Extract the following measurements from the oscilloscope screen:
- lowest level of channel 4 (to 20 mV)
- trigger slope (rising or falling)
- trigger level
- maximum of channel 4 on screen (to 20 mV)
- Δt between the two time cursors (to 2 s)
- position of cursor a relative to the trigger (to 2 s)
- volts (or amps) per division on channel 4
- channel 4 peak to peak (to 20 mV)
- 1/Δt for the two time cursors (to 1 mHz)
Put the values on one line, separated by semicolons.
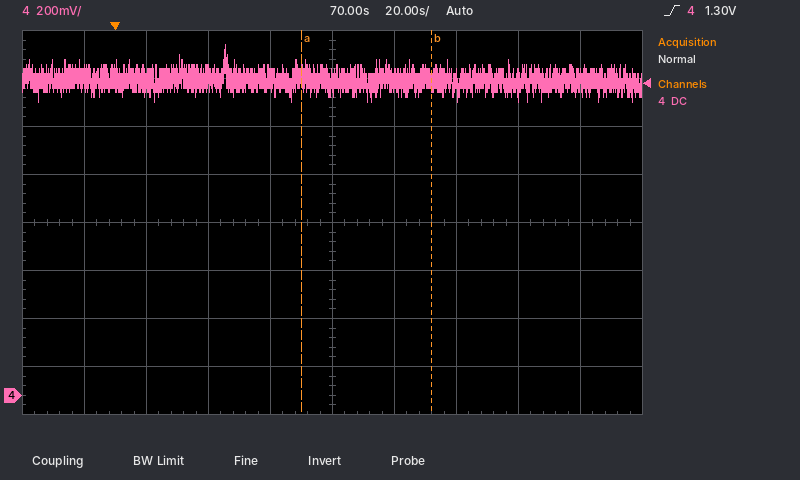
1.22 V; rising; 1.30 V; 1.46 V; 42 s; +60 s; 200 mV; 240 mV; 24 mHz
